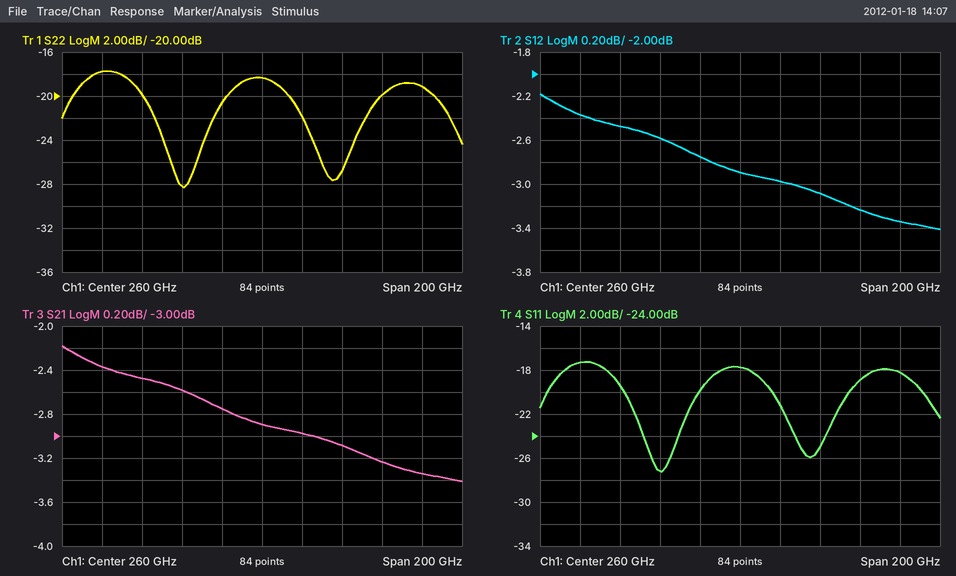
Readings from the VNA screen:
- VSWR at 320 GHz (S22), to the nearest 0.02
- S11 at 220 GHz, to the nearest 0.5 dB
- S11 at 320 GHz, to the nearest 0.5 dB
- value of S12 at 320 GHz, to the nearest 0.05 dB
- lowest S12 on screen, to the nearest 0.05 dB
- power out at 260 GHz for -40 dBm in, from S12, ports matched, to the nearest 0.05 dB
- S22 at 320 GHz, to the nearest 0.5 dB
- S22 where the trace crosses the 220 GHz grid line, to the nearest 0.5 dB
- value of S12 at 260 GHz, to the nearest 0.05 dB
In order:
1.22
-27.0 dB
-19.0 dB
-3.25 dB
-3.40 dB
-42.90 dBm
-20.0 dB
-28.0 dB
-2.90 dB
